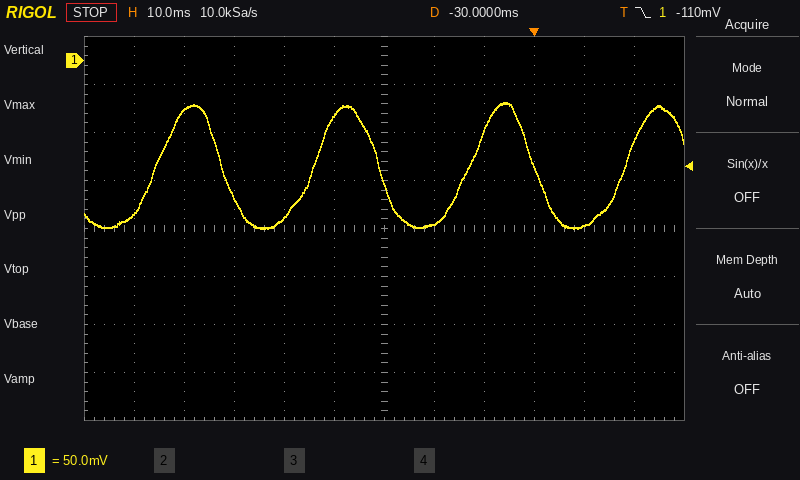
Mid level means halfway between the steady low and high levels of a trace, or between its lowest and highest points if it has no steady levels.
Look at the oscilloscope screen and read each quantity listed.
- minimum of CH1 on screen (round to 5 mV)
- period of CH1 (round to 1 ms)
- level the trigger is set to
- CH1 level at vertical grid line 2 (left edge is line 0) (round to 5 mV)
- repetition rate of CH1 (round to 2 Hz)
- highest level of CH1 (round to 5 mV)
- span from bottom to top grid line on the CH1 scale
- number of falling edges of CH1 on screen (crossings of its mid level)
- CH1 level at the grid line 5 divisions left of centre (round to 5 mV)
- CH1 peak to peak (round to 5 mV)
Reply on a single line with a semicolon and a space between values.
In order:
-175 mV; 31 ms; -110 mV; -50 mV; 32 Hz; -45 mV; 400 mV; 3; -160 mV; 130 mV
